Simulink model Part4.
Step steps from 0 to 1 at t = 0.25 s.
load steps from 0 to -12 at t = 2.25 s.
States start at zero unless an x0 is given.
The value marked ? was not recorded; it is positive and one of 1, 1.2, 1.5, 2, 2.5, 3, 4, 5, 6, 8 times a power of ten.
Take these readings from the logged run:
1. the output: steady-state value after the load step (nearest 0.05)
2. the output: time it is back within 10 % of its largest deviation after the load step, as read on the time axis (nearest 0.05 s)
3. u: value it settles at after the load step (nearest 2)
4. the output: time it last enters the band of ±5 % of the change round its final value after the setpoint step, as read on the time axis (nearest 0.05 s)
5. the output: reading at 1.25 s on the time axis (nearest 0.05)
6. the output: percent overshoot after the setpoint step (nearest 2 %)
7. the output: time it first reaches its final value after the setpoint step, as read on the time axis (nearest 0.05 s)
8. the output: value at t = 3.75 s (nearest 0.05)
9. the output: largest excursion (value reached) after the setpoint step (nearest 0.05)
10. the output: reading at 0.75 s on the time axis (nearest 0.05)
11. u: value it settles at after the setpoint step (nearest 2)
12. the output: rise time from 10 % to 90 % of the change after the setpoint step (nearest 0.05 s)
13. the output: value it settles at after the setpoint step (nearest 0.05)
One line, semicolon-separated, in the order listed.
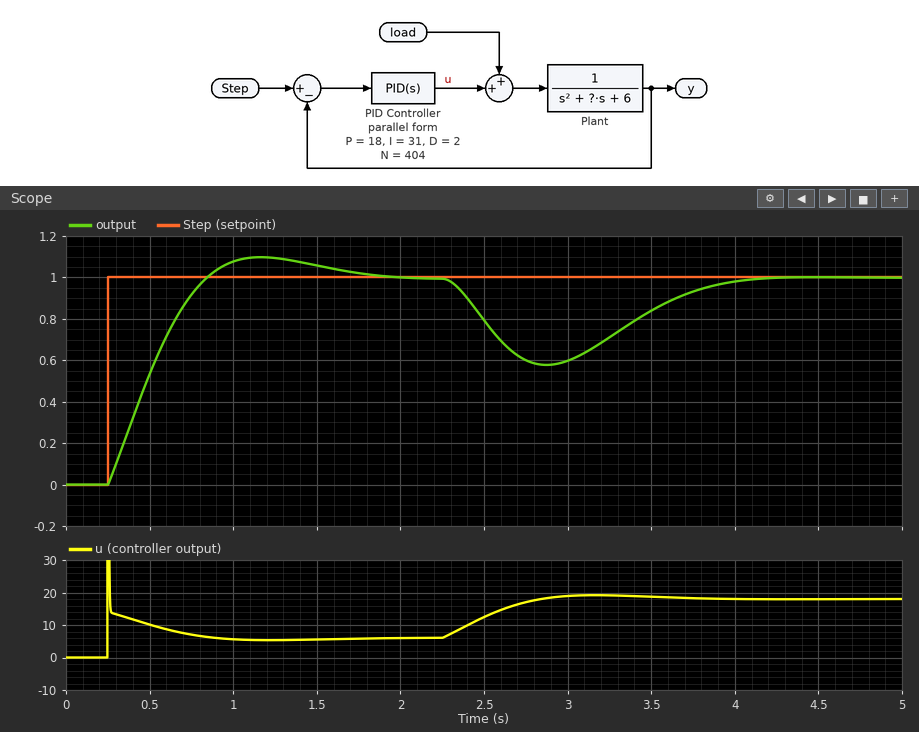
1.00; 3.85 s; 18; 1.55 s; 1.10; 10 %; 0.85 s; 0.95; 1.10; 0.90; 6; 0.45 s; 1.00
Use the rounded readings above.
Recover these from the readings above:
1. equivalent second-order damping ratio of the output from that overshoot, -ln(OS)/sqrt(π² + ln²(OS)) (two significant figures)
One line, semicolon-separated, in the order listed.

0.59
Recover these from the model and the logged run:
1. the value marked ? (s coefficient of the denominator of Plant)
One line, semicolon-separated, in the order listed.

5
